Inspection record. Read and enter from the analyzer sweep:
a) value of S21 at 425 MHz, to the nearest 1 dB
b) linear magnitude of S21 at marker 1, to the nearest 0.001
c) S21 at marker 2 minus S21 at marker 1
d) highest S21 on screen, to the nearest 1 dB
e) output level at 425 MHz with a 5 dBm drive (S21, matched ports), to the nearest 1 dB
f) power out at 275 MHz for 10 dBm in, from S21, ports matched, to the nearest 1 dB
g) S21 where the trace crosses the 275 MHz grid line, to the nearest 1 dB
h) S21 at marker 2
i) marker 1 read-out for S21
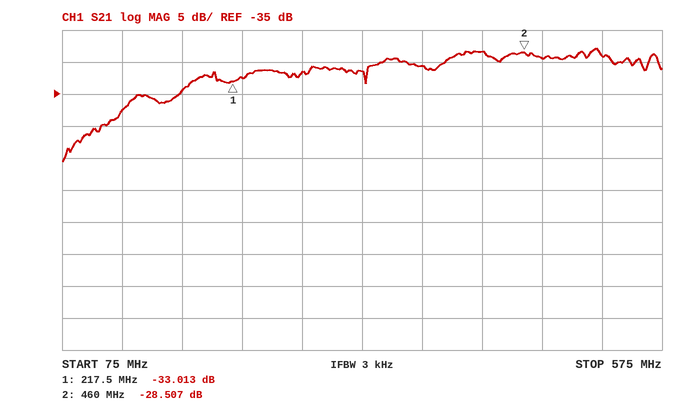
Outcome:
-28 dB
0.022
4.506 dB
-28 dB
-23 dBm
-22 dBm
-32 dB
-28.507 dB
-33.013 dB
